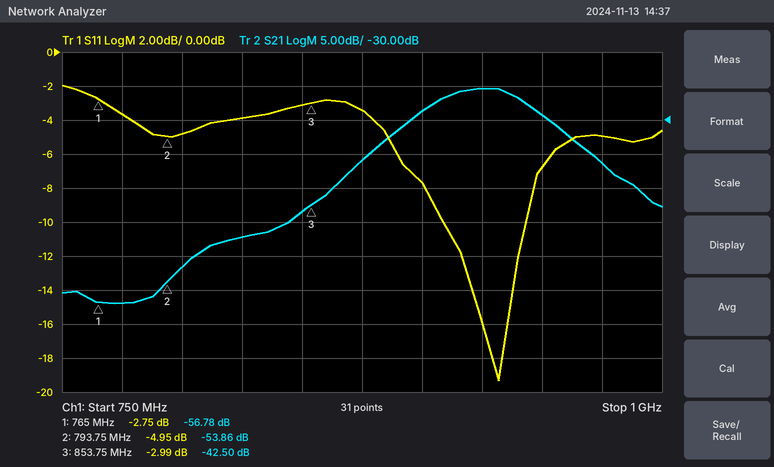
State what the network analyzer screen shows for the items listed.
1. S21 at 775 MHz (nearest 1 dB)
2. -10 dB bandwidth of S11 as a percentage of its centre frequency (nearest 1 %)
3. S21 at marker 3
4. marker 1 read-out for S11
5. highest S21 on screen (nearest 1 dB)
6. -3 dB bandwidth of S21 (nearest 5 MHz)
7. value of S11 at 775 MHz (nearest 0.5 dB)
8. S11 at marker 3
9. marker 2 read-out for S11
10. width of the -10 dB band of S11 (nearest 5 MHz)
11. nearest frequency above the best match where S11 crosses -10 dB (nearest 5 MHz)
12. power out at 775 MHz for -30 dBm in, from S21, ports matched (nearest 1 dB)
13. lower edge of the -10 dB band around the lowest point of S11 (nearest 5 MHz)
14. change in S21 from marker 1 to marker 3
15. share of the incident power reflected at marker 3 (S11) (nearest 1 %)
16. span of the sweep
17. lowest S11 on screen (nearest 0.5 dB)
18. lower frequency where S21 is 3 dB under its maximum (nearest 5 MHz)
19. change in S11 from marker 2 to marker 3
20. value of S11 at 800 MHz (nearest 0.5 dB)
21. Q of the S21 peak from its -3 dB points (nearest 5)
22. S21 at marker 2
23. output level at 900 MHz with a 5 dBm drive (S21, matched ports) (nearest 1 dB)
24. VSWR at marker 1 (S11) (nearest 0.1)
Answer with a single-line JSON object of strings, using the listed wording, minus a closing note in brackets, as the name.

{"S21 at 775 MHz": "-57 dB", "-10 dB bandwidth of S11 as a percentage of its centre frequency": "4 %", "S21 at marker 3": "-42.50 dB", "marker 1 read-out for S11": "-2.75 dB", "highest S21 on screen": "-25 dB", "-3 dB bandwidth of S21": "45 MHz", "value of S11 at 775 MHz": "-3.5 dB", "S11 at marker 3": "-2.99 dB", "marker 2 read-out for S11": "-4.95 dB", "width of the -10 dB band of S11": "35 MHz", "nearest frequency above the best match where S11 crosses -10 dB": "945 MHz", "power out at 775 MHz for -30 dBm in, from S21, ports matched": "-87 dBm", "lower edge of the -10 dB band around the lowest point of S11": "910 MHz", "change in S21 from marker 1 to marker 3": "14.28 dB", "share of the incident power reflected at marker 3 (S11)": "50 %", "span of the sweep": "250 MHz", "lowest S11 on screen": "-19.5 dB", "lower frequency where S21 is 3 dB under its maximum": "900 MHz", "change in S11 from marker 2 to marker 3": "1.96 dB", "value of S11 at 800 MHz": "-5.0 dB", "Q of the S21 peak from its -3 dB points": "20", "S21 at marker 2": "-53.86 dB", "output level at 900 MHz with a 5 dBm drive (S21, matched ports)": "-24 dBm", "VSWR at marker 1 (S11)": "6.4"}
